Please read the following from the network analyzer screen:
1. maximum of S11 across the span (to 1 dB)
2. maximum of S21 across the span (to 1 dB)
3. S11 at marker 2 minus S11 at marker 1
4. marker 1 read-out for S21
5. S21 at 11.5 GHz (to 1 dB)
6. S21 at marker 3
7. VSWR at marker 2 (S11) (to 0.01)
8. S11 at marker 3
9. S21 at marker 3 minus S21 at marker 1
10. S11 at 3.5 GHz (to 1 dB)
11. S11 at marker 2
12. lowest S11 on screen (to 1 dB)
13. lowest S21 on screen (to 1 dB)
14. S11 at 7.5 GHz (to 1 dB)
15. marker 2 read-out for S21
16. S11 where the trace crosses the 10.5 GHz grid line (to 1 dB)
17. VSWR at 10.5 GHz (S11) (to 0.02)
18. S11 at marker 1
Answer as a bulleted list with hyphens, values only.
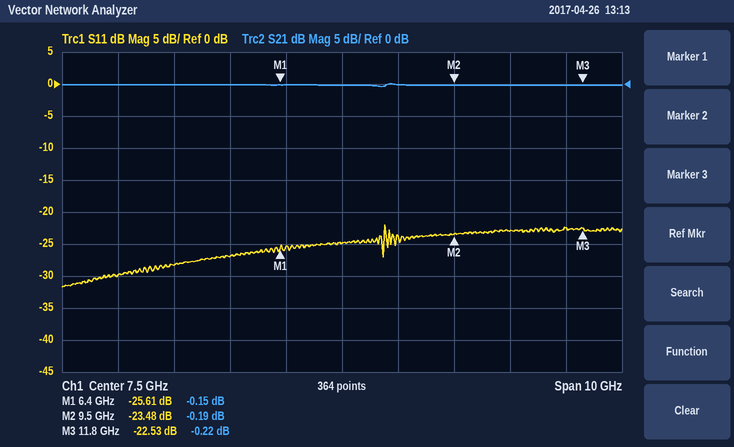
- -22 dB
- 0 dB
- 2.13 dB
- -0.15 dB
- 0 dB
- -0.22 dB
- 1.14
- -22.53 dB
- -0.07 dB
- -30 dB
- -23.48 dB
- -32 dB
- 0 dB
- -25 dB
- -0.19 dB
- -23 dB
- 1.16
- -25.61 dB
